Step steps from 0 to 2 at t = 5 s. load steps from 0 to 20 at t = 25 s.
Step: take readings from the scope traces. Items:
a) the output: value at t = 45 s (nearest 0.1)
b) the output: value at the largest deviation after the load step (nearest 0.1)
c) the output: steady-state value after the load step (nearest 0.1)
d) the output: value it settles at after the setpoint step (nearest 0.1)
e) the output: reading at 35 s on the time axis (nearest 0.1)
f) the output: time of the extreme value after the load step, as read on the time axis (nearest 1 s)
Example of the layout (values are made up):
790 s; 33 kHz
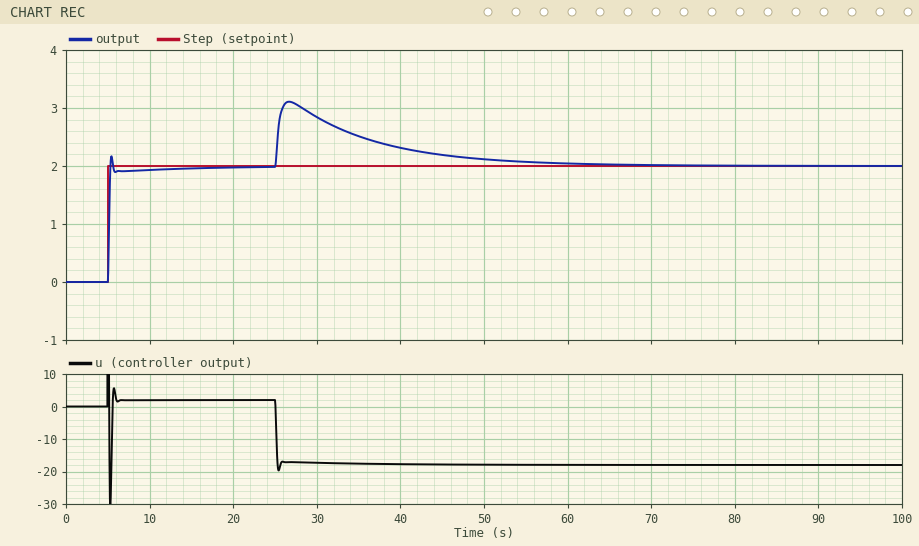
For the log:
2.2; 3.1; 2.0; 2.0; 2.5; 27 s
